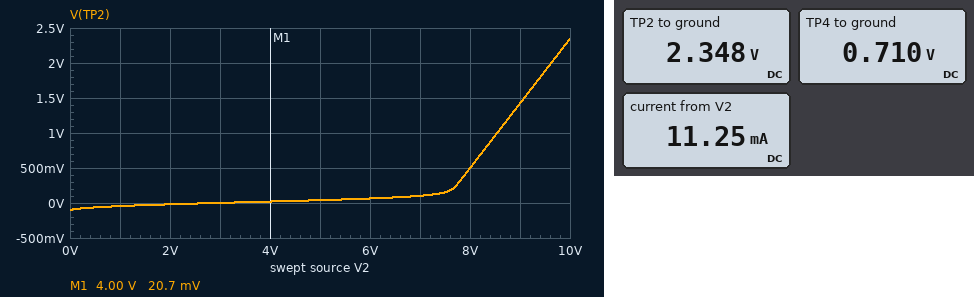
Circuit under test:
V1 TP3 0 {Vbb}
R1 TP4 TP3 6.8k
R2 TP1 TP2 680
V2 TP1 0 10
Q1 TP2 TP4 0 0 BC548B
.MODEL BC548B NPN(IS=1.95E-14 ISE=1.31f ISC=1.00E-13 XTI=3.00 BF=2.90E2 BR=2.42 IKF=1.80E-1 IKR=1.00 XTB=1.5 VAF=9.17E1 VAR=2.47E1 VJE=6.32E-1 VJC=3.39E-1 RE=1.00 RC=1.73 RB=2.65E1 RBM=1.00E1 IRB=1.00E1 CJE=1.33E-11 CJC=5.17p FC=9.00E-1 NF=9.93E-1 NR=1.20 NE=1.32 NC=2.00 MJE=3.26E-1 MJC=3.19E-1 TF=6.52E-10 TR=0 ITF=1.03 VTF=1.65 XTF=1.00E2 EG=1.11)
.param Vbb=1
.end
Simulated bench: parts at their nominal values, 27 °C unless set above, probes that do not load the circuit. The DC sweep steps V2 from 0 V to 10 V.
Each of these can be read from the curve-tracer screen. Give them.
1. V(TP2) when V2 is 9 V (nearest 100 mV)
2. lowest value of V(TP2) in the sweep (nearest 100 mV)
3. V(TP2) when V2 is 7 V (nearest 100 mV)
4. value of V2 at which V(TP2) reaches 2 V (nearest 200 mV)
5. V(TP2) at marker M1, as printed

1.4 V
-100 mV
100 mV
9.6 V
20.7 mV
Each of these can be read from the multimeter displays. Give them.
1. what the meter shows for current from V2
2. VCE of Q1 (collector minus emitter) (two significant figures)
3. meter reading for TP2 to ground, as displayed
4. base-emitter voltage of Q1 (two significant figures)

11.25 mA
2.3 V
2.348 V
710 mV
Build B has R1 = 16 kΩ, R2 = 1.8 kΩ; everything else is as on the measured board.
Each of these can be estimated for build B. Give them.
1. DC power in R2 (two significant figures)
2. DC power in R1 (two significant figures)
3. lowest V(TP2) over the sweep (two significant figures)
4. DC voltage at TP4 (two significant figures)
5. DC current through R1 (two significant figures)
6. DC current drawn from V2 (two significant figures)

50 mW
6.3 µW
-95 mV
680 mV
20 µA
5.3 mA
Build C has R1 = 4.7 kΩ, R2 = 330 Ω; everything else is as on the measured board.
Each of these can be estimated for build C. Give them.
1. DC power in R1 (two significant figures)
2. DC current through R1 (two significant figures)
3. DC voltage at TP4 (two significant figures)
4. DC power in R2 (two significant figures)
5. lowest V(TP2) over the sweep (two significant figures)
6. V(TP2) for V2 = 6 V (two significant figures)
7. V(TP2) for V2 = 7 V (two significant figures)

16 µW
59 µA
720 mV
81 mW
-94 mV
1.0 V
2.0 V
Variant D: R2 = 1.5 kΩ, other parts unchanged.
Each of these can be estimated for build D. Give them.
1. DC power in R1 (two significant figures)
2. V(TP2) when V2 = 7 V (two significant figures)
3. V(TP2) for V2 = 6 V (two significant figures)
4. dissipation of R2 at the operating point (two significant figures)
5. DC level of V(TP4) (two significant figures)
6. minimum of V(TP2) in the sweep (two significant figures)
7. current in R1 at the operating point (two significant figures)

14 µW
5.0 mV
-3.9 mV
66 mW
690 mV
-100 mV
45 µA
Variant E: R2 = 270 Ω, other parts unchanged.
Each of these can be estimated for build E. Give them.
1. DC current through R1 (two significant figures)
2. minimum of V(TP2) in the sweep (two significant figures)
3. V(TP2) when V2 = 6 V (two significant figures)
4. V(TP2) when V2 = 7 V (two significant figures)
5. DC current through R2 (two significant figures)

43 µA
-85 mV
2.9 V
3.9 V
12 mA
